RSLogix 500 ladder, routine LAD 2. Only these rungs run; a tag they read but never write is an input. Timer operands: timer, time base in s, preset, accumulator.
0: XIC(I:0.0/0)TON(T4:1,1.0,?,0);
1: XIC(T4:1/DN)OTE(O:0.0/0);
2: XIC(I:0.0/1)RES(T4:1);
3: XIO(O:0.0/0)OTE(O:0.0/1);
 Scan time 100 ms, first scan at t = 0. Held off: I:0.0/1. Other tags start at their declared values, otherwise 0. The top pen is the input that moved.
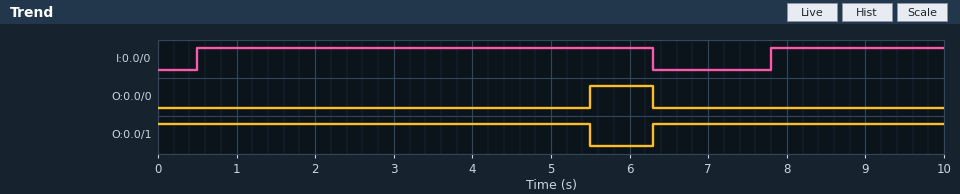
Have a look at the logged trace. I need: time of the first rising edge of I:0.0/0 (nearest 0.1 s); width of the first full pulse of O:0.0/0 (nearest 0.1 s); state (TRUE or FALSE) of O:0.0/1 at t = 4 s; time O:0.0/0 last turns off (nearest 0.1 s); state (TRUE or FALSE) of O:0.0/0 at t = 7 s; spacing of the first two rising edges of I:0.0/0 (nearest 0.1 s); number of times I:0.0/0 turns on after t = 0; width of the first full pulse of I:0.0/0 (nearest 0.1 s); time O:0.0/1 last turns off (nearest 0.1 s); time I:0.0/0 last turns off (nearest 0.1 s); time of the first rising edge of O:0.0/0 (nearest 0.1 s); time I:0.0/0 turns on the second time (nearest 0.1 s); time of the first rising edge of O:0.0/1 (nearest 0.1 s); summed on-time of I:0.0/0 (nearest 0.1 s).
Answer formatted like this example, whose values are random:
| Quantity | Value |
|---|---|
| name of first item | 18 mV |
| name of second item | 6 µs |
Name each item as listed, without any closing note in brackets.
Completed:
| Quantity | Value |
|---|---|
| time of the first rising edge of I:0.0/0 | 0.5 s |
| width of the first full pulse of O:0.0/0 | 0.8 s |
| state (TRUE or FALSE) of O:0.0/1 at t = 4 s | TRUE |
| time O:0.0/0 last turns off | 6.3 s |
| state (TRUE or FALSE) of O:0.0/0 at t = 7 s | FALSE |
| spacing of the first two rising edges of I:0.0/0 | 7.3 s |
| number of times I:0.0/0 turns on after t = 0 | 2 |
| width of the first full pulse of I:0.0/0 | 5.8 s |
| time O:0.0/1 last turns off | 5.5 s |
| time I:0.0/0 last turns off | 6.3 s |
| time of the first rising edge of O:0.0/0 | 5.5 s |
| time I:0.0/0 turns on the second time | 7.8 s |
| time of the first rising edge of O:0.0/1 | 6.3 s |
| summed on-time of I:0.0/0 | 8.0 s |
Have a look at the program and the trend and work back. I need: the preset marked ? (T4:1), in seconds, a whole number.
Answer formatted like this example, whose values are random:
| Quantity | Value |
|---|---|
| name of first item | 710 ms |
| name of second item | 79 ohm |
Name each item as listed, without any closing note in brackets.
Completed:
| Quantity | Value |
|---|---|
| the preset marked ? (T4:1), in seconds, a whole number | 5 s |
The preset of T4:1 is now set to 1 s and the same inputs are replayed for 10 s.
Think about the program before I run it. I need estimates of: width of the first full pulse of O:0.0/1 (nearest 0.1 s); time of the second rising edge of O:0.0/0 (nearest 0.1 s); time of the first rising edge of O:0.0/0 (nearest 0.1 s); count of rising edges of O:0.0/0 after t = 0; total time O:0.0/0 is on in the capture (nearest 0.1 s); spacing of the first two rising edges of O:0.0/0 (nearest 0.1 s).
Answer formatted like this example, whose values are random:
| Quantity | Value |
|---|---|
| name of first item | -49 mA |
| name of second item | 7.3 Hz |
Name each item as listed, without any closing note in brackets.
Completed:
| Quantity | Value |
|---|---|
| width of the first full pulse of O:0.0/1 | 2.5 s |
| time of the second rising edge of O:0.0/0 | 8.8 s |
| time of the first rising edge of O:0.0/0 | 1.5 s |
| count of rising edges of O:0.0/0 after t = 0 | 2 |
| total time O:0.0/0 is on in the capture | 6.0 s |
| spacing of the first two rising edges of O:0.0/0 | 7.3 s |
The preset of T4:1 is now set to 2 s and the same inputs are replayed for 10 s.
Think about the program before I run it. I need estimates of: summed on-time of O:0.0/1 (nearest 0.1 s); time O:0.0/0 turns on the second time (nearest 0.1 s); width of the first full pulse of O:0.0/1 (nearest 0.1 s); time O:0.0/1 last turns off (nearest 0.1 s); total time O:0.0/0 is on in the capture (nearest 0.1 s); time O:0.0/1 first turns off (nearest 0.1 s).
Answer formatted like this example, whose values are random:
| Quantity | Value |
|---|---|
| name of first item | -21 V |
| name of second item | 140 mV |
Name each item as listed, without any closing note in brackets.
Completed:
| Quantity | Value |
|---|---|
| summed on-time of O:0.0/1 | 6.0 s |
| time O:0.0/0 turns on the second time | 9.8 s |
| width of the first full pulse of O:0.0/1 | 3.5 s |
| time O:0.0/1 last turns off | 9.8 s |
| total time O:0.0/0 is on in the capture | 4.0 s |
| time O:0.0/1 first turns off | 2.5 s |
